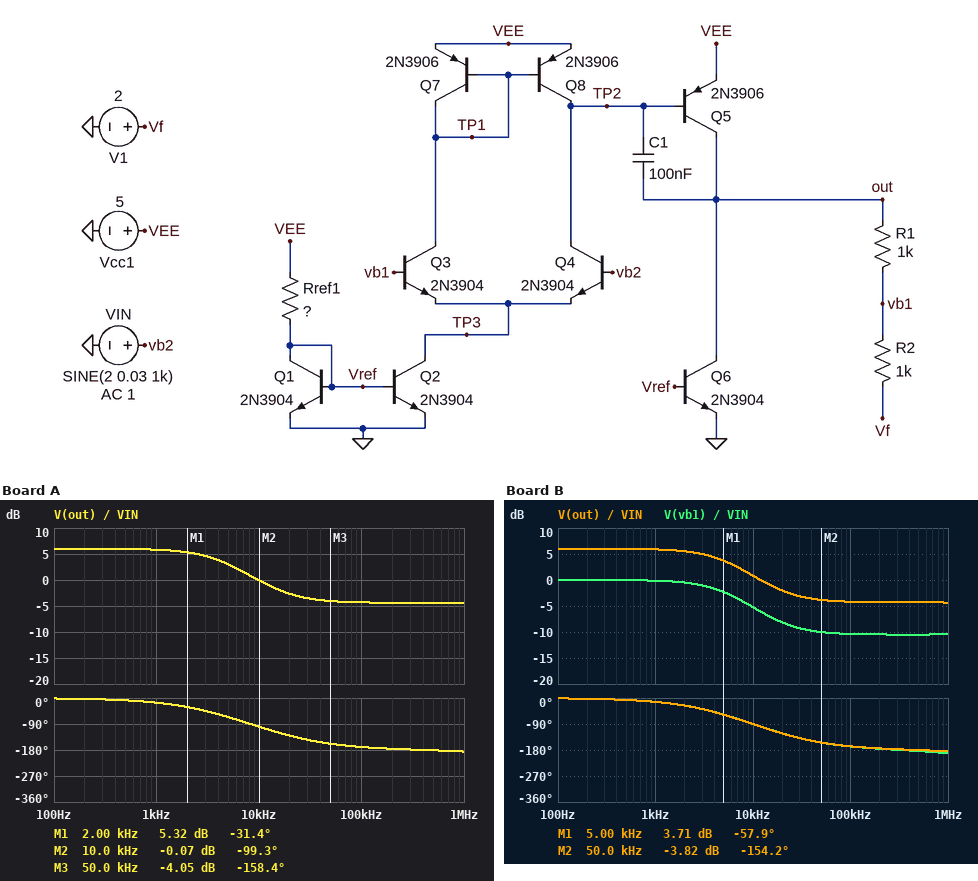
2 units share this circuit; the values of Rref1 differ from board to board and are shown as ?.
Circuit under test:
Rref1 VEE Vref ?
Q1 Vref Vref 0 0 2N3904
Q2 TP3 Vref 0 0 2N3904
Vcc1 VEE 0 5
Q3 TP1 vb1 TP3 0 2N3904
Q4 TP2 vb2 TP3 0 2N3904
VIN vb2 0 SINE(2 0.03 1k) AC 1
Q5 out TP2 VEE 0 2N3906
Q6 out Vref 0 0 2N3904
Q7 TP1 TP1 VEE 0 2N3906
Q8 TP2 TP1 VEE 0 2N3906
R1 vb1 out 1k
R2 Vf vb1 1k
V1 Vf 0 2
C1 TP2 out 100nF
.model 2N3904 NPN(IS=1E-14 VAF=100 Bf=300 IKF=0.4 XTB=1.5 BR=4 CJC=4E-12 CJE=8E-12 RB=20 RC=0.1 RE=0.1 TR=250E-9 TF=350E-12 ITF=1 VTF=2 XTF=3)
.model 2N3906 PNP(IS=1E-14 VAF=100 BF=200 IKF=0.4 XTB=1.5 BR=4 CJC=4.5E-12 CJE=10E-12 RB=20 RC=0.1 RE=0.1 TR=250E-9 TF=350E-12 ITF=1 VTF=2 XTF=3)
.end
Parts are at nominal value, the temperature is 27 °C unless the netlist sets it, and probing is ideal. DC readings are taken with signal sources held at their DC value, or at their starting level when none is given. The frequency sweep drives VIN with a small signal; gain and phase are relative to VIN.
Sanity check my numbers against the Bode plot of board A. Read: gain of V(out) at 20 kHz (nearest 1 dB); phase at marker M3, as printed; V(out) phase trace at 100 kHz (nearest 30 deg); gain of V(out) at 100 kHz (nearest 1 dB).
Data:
-3 dB
-158.4 deg
-180 deg
-4 dB
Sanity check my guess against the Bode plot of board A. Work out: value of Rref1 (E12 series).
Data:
18 kΩ
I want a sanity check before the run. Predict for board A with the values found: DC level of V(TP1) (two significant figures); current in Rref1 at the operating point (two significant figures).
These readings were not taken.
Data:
4.4 V
240 µA
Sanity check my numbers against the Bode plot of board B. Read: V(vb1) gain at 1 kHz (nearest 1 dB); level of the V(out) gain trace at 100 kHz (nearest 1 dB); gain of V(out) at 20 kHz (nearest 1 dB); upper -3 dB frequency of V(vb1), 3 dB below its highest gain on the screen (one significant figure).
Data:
0 dB
-4 dB
-2 dB
6 kHz
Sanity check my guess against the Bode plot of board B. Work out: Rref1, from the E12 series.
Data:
15 kΩ
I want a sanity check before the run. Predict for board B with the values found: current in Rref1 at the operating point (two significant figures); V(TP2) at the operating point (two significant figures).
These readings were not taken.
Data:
290 µA
4.4 V
